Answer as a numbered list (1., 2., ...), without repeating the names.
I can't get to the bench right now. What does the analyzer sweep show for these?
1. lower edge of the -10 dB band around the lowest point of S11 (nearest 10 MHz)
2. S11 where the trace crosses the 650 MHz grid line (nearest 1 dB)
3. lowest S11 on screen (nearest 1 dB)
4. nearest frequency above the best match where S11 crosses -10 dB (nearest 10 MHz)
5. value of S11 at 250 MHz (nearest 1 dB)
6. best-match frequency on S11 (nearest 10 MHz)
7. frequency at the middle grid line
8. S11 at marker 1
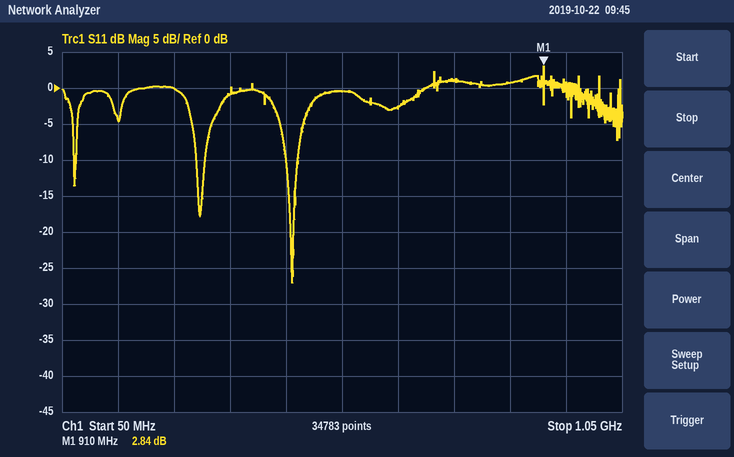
1. 450 MHz
2. -3 dB
3. -27 dB
4. 470 MHz
5. 0 dB
6. 460 MHz
7. 550 MHz
8. 2.84 dB
